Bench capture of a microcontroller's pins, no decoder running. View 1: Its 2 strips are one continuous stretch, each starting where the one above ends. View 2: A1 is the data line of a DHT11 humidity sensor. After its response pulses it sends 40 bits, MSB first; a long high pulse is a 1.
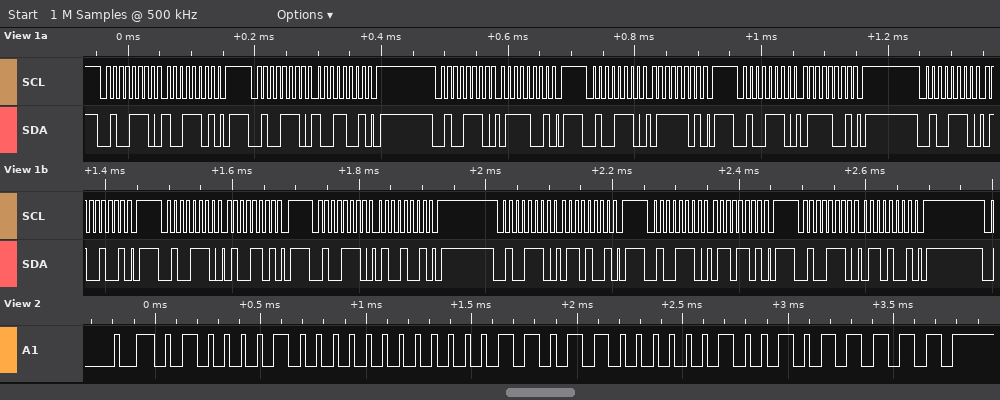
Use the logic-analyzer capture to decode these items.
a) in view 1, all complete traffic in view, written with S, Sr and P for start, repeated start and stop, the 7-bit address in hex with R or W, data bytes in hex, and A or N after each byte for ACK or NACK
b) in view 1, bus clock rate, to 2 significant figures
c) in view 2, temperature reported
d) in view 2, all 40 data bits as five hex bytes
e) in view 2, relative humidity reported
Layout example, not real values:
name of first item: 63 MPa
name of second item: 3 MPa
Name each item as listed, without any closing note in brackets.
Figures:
in view 1, all complete traffic in view, written with S, Sr and P for start, repeated start and stop, the 7-bit address in hex with R or W, data bytes in hex, and A or N after each byte for ACK or NACK: S 27W A 9D A P S 27W A 99 A P S 27W A 79 A P S 27W A 7D A P S 27W A 79 A P S 27W A 49 A P S 27W A 4D A P S 27W A 49 A P S 27W A 69 A P S 27W A 6D A P S 27W A 69 A P
in view 1, bus clock rate, to 2 significant figures: 100 kHz
in view 2, temperature reported: 27.2 °C
in view 2, all 40 data bits as five hex bytes: 42 00 1B 02 5F
in view 2, relative humidity reported: 66 %
